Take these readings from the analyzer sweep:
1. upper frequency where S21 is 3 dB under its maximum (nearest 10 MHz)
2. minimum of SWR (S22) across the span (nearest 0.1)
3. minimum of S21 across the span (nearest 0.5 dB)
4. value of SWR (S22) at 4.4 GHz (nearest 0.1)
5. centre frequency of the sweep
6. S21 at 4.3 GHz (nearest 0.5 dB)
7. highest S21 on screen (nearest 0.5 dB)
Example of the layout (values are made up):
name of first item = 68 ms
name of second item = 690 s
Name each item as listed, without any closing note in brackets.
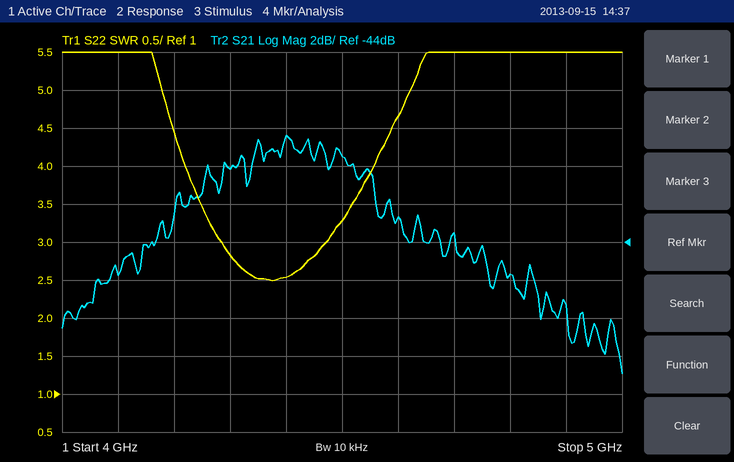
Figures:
upper frequency where S21 is 3 dB under its maximum = 4.56 GHz
minimum of SWR (S22) across the span = 2.5
minimum of S21 across the span = -51.0 dB
value of SWR (S22) at 4.4 GHz = 2.5
centre frequency of the sweep = 4.5 GHz
S21 at 4.3 GHz = -40.0 dB
highest S21 on screen = -38.5 dB
